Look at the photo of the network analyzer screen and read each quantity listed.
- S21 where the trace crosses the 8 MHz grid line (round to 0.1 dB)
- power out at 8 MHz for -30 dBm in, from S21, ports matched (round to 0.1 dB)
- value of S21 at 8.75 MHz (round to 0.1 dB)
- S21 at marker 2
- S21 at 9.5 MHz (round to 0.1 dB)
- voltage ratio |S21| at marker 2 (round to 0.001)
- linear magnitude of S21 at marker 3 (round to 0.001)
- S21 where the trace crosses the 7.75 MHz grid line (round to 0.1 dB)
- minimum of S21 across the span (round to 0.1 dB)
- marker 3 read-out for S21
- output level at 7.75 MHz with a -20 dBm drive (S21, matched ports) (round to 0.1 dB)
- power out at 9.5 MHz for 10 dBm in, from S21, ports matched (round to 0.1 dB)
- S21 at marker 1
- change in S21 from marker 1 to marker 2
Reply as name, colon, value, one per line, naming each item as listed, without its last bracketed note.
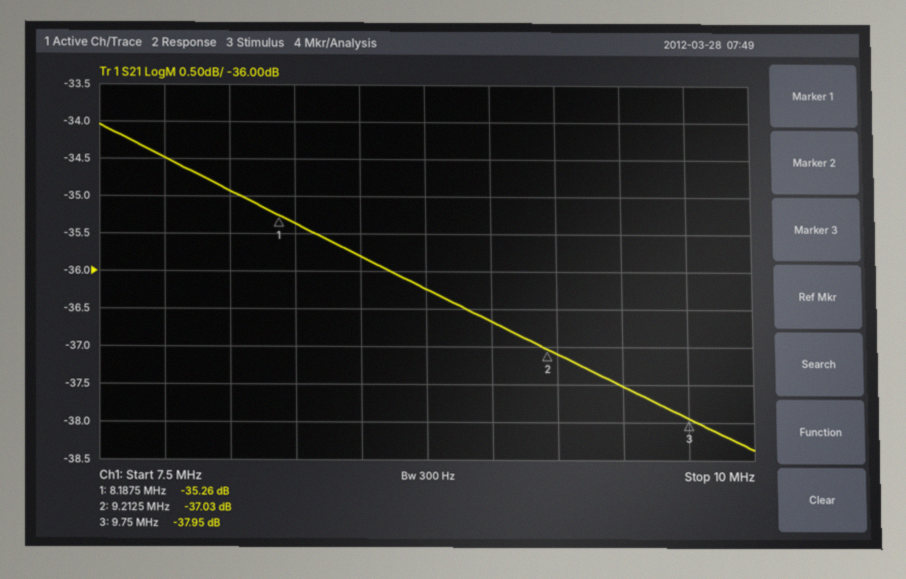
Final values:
S21 where the trace crosses the 8 MHz grid line: -34.9 dB
power out at 8 MHz for -30 dBm in, from S21, ports matched: -64.9 dBm
value of S21 at 8.75 MHz: -36.2 dB
S21 at marker 2: -37.03 dB
S21 at 9.5 MHz: -37.5 dB
voltage ratio |S21| at marker 2: 0.014
linear magnitude of S21 at marker 3: 0.013
S21 where the trace crosses the 7.75 MHz grid line: -34.5 dB
minimum of S21 across the span: -38.4 dB
marker 3 read-out for S21: -37.95 dB
output level at 7.75 MHz with a -20 dBm drive (S21, matched ports): -54.5 dBm
power out at 9.5 MHz for 10 dBm in, from S21, ports matched: -27.5 dBm
S21 at marker 1: -35.26 dB
change in S21 from marker 1 to marker 2: -1.77 dB
